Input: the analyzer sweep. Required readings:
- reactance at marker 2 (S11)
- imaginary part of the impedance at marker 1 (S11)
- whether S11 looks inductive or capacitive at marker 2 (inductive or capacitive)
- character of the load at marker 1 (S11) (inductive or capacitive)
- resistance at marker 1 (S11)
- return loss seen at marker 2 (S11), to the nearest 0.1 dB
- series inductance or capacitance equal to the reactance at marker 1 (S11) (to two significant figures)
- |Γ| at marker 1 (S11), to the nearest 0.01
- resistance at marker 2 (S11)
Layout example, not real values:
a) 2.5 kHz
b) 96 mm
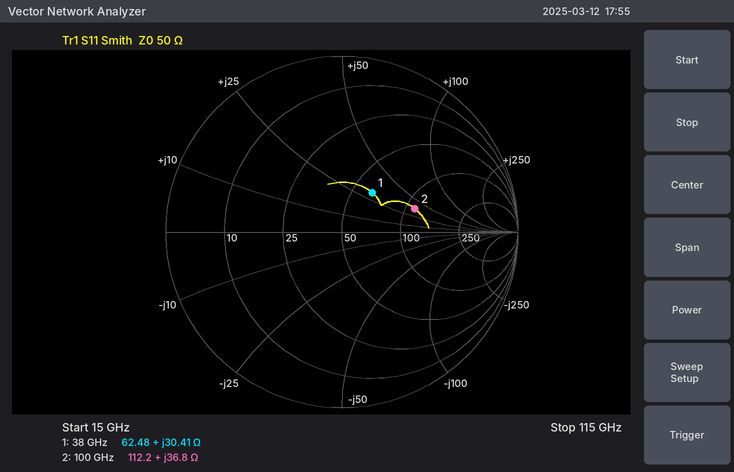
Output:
a) +36.8 Ω
b) +30.41 Ω
c) inductive
d) inductive
e) 62.48 Ω
f) 7.2 dB
g) 130 pH
h) 0.28
i) 112.2 Ω
